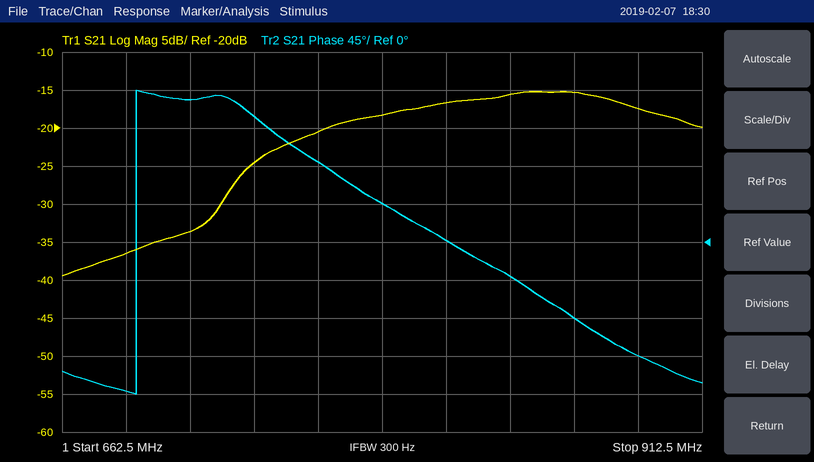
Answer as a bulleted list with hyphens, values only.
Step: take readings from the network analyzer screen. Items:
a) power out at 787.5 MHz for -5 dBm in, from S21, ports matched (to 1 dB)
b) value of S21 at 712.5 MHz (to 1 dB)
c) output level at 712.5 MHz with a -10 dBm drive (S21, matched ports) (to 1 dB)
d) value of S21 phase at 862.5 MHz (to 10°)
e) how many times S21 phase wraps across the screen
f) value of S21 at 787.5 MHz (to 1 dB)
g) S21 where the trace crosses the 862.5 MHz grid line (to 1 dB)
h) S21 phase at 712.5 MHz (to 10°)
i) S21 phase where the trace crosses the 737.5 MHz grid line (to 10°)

- -23 dBm
- -34 dB
- -44 dBm
- -90°
- 1
- -18 dB
- -15 dB
- 170°
- 150°
